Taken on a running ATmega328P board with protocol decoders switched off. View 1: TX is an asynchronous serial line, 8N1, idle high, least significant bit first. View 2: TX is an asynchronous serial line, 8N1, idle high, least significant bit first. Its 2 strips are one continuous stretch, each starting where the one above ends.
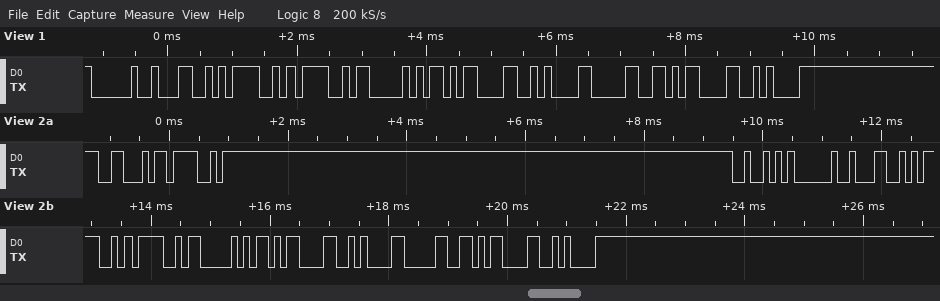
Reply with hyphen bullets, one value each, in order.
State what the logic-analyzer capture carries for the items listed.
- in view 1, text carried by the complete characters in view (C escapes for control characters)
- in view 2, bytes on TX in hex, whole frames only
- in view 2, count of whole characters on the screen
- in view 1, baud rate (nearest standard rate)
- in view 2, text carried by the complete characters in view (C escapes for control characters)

- " LOOP\r\n0\r\n"
- 0x46 0x4F 0x52 0x20 0x4C 0x4F 0x4F 0x50 0x0D 0x0A 0x30 0x0D 0x0A
- 13
- 9600 baud
- "FOR LOOP\r\n0\r\n"
